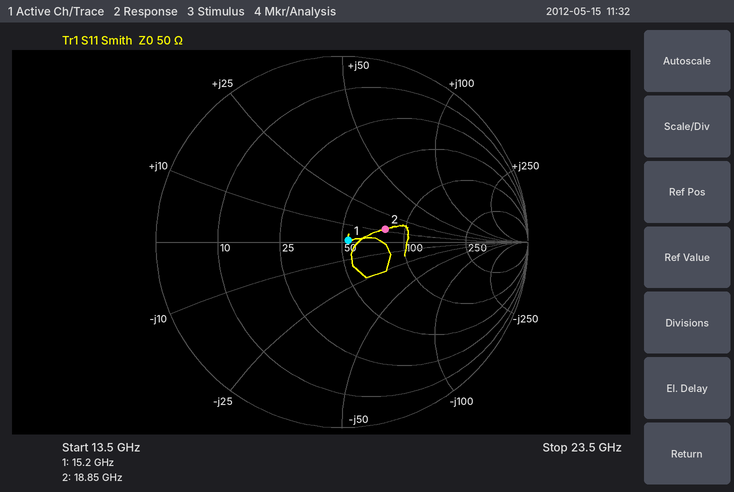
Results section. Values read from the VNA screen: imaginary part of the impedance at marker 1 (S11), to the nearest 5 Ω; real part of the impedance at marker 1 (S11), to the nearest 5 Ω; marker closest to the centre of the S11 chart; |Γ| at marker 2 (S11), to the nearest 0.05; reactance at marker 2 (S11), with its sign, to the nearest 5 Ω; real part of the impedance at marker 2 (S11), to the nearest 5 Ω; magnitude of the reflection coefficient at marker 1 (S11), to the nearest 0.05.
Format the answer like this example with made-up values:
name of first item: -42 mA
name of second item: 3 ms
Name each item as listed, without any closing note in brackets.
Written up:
imaginary part of the impedance at marker 1 (S11), to the nearest 5 Ω: 0 Ω
real part of the impedance at marker 1 (S11), to the nearest 5 Ω: 55 Ω
marker closest to the centre of the S11 chart: marker 1
|Γ| at marker 2 (S11), to the nearest 0.05: 0.25
reactance at marker 2 (S11), with its sign, to the nearest 5 Ω: +10 Ω
real part of the impedance at marker 2 (S11), to the nearest 5 Ω: 80 Ω
magnitude of the reflection coefficient at marker 1 (S11), to the nearest 0.05: 0.05
